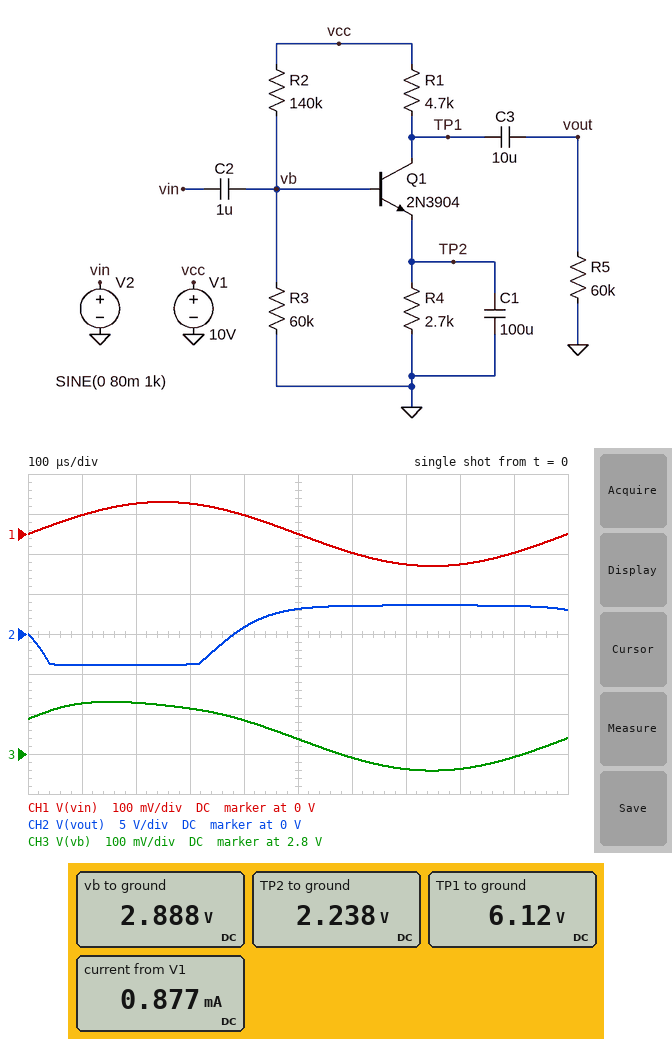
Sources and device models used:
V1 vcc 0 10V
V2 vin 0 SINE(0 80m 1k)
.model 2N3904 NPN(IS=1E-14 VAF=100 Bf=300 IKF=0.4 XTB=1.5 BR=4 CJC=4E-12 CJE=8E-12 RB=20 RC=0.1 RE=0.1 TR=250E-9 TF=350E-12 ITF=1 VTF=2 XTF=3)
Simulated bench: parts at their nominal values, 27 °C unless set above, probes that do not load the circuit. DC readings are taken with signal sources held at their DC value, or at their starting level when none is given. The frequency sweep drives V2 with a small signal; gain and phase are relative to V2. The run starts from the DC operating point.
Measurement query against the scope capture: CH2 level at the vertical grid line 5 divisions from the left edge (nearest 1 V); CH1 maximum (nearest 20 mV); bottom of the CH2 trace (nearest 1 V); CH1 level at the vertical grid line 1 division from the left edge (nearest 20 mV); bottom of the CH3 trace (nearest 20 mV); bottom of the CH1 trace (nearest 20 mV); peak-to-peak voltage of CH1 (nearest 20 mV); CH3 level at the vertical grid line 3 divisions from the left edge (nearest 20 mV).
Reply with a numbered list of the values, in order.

1. 3 V
2. 80 mV
3. -4 V
4. 40 mV
5. 2.76 V
6. -80 mV
7. 160 mV
8. 2.92 V
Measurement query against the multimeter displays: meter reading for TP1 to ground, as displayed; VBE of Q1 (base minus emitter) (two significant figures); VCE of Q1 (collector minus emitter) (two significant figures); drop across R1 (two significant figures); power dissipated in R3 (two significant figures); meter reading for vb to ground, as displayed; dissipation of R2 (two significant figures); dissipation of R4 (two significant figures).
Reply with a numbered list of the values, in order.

1. 6.12 V
2. 650 mV
3. 3.9 V
4. 3.9 V
5. 140 µW
6. 2.888 V
7. 360 µW
8. 1.9 mW
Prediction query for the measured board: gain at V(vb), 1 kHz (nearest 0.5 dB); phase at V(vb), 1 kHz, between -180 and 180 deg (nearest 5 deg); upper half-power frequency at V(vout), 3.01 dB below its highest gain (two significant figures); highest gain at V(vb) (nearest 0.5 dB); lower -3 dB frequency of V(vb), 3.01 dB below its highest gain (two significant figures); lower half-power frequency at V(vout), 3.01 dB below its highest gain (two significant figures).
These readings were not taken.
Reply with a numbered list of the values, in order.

1. 0 dB
2. 0 deg
3. 9.9 MHz
4. 0 dB
5. 8.7 Hz
6. 67 Hz
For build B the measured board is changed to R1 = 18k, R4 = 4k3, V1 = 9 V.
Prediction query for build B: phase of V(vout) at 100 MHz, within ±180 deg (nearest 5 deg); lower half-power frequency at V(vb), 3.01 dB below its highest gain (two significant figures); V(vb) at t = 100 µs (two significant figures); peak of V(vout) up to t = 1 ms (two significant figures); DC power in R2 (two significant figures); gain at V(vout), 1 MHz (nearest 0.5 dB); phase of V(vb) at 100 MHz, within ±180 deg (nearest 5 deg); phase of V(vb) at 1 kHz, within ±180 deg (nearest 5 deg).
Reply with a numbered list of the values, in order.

1. -5 deg
2. 490 Hz
3. 2.4 V
4. 5.5 V
5. 310 µW
6. 16.0 dB
7. 0 deg
8. 25 deg
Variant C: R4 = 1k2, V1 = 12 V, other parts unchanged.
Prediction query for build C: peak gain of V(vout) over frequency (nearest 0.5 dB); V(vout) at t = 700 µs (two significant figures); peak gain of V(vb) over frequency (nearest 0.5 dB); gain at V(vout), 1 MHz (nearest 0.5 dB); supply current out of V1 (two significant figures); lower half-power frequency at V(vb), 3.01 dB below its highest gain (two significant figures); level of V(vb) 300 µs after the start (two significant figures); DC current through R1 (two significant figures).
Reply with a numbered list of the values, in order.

1. 34.0 dB
2. 8.7 V
3. 0 dB
4. 26.5 dB
5. 2.1 mA
6. 1.7 kHz
7. 3.1 V
8. 2.0 mA
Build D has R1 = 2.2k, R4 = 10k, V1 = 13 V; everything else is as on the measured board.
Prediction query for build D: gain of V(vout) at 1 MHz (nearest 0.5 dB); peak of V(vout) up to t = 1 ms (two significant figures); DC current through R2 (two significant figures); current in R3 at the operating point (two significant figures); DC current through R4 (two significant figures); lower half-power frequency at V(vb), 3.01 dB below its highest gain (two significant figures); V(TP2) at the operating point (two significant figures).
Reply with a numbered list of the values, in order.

1. 28.5 dB
2. 670 mV
3. 65 µA
4. 64 µA
5. 320 µA
6. 7.3 Hz
7. 3.2 V
